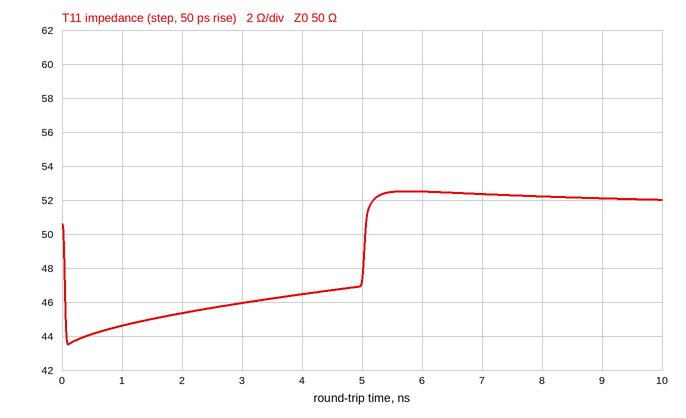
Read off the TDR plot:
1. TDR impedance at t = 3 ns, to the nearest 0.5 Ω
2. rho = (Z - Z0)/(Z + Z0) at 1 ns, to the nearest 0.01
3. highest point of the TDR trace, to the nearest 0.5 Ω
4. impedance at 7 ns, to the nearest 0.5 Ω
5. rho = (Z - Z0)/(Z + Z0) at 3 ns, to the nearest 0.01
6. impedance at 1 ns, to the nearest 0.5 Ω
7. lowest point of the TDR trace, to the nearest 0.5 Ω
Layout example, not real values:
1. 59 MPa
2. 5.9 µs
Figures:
1. 46.0 Ω
2. -0.06
3. 52.5 Ω
4. 52.5 Ω
5. -0.04
6. 44.5 Ω
7. 43.5 Ω
